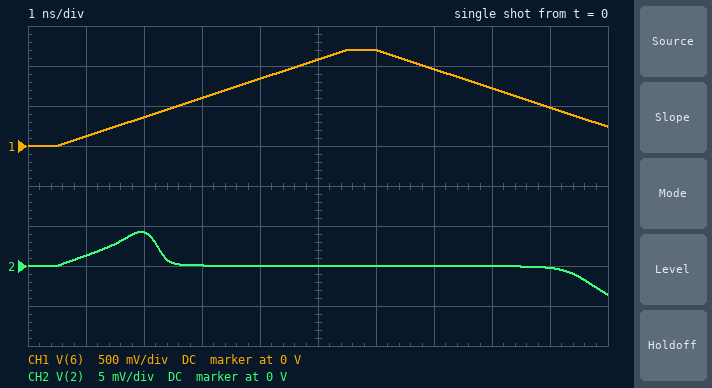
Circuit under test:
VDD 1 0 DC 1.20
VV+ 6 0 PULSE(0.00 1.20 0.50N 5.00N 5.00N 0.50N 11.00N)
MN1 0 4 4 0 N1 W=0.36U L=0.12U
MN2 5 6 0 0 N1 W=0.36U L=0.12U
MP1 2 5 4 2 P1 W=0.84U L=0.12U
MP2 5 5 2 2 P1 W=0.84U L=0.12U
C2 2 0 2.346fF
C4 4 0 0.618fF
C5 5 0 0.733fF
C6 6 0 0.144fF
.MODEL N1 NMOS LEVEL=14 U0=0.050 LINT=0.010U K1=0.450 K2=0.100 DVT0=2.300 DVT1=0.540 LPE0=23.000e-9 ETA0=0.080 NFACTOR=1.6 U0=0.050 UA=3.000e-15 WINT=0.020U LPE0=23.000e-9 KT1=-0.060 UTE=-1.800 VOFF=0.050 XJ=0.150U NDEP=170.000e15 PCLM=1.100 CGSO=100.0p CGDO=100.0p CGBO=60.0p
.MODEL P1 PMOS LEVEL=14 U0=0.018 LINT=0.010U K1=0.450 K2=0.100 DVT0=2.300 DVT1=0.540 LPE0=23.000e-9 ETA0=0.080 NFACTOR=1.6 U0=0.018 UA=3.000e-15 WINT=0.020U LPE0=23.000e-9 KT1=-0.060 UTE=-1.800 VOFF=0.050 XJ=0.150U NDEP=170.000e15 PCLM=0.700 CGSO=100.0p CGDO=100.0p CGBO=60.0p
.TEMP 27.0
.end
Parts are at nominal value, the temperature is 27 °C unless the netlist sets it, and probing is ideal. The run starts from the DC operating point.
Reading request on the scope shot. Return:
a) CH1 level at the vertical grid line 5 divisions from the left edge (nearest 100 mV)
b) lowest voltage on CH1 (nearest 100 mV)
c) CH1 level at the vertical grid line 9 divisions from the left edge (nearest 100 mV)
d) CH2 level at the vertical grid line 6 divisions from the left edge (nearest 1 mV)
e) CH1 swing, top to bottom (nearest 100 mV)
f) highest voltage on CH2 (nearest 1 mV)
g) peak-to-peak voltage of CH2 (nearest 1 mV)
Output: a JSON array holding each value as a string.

["1.1 V", "0 V", "500 mV", "0 V", "1.2 V", "4 mV", "8 mV"]
